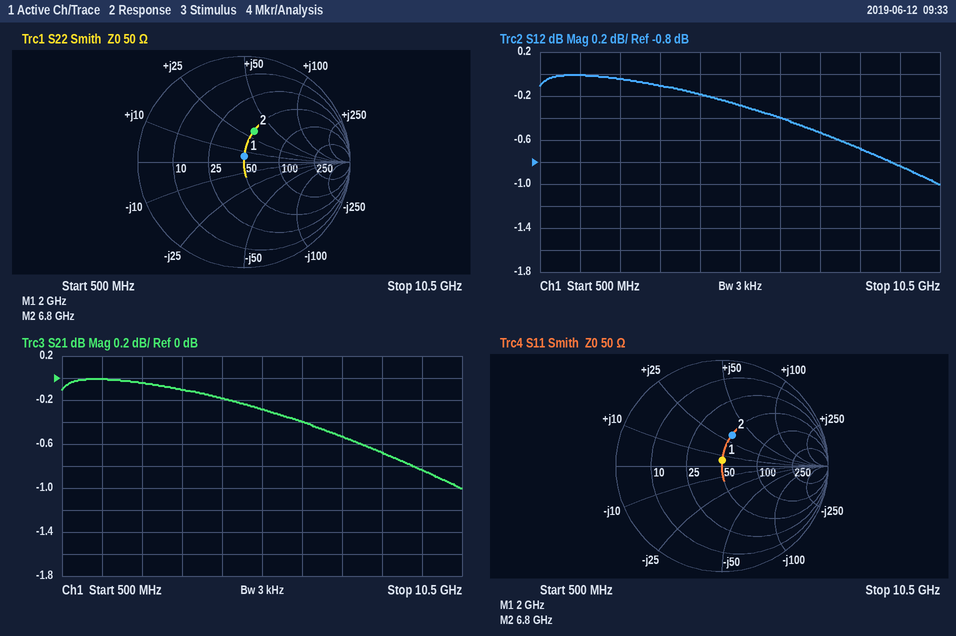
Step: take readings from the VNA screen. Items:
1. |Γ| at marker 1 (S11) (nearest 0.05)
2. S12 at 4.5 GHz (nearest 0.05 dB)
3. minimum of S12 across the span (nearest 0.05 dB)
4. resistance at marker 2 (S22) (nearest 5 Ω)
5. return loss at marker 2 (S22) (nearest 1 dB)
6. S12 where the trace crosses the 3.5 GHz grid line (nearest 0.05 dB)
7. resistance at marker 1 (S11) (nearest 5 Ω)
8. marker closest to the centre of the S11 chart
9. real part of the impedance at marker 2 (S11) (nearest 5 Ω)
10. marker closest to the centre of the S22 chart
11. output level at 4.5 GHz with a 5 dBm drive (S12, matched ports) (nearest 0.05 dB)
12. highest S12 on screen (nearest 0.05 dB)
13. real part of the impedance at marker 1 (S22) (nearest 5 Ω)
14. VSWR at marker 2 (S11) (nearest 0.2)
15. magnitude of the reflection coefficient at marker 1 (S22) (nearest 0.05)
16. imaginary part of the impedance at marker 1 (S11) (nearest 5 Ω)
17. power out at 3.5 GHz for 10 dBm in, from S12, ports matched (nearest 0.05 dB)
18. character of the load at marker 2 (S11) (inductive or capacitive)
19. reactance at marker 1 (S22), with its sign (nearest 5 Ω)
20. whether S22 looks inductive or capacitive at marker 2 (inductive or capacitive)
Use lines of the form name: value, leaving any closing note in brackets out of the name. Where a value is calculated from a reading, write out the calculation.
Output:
|Γ| at marker 1 (S11): 0.05
S12 at 4.5 GHz: -0.20 dB
minimum of S12 across the span: -1.00 dB
resistance at marker 2 (S22): 50 Ω
return loss at marker 2 (S22): 10 dB
S12 where the trace crosses the 3.5 GHz grid line: -0.10 dB
resistance at marker 1 (S11): 50 Ω
marker closest to the centre of the S11 chart: marker 1
real part of the impedance at marker 2 (S11): 50 Ω
marker closest to the centre of the S22 chart: marker 1
output level at 4.5 GHz with a 5 dBm drive (S12, matched ports): 5 dBm + (-0.20 dB) = 4.80 dBm
highest S12 on screen: 0.00 dB
real part of the impedance at marker 1 (S22): 50 Ω
VSWR at marker 2 (S11): 1.8
magnitude of the reflection coefficient at marker 1 (S22): 0.05
imaginary part of the impedance at marker 1 (S11): +5 Ω
power out at 3.5 GHz for 10 dBm in, from S12, ports matched: 10 dBm + (-0.10 dB) = 9.90 dBm
character of the load at marker 2 (S11): inductive
reactance at marker 1 (S22), with its sign: +5 Ω
whether S22 looks inductive or capacitive at marker 2: inductive
